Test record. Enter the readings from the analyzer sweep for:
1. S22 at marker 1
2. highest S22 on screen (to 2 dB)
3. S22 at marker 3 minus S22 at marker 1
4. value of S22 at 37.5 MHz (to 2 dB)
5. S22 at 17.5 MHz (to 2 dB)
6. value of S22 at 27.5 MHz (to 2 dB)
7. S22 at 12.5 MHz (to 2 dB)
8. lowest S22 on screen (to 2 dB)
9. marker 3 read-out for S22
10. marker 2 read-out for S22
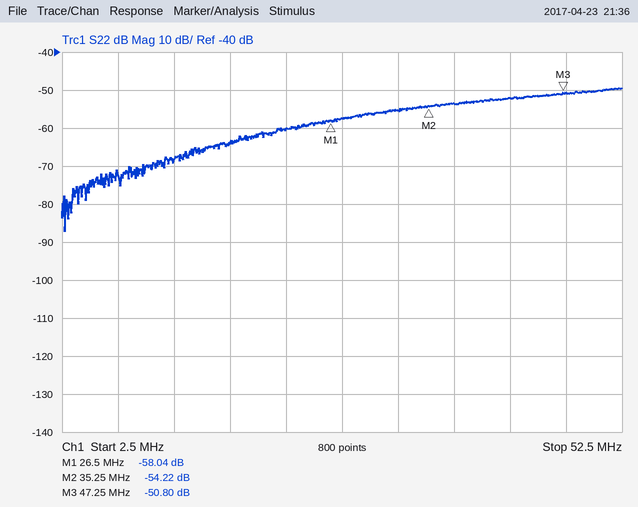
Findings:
-58.04 dB
-50 dB
7.24 dB
-54 dB
-64 dB
-58 dB
-68 dB
-88 dB
-50.80 dB
-54.22 dB
